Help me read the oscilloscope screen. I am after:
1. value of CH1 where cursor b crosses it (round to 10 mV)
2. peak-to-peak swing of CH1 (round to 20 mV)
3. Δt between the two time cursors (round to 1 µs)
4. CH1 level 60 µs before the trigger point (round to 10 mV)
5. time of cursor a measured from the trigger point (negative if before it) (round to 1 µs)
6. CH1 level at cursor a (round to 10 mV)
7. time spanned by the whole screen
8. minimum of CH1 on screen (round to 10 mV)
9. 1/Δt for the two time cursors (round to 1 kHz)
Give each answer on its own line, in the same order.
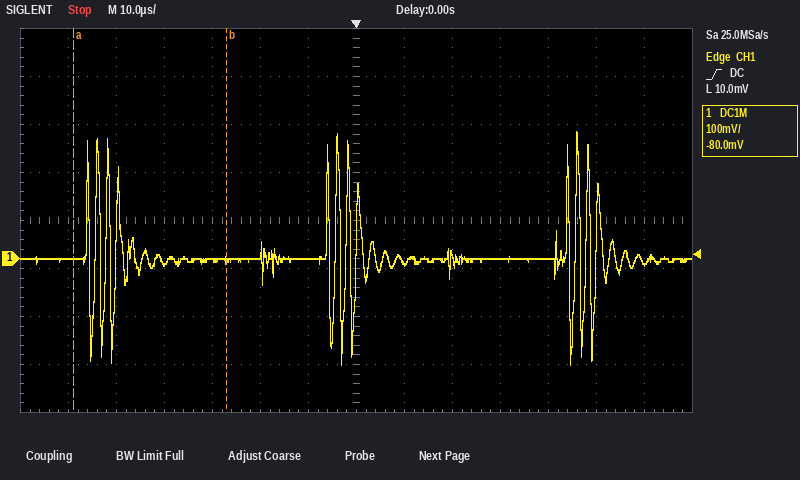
0 mV
480 mV
32 µs
0 mV
-59 µs
0 mV
140 µs
-220 mV
31 kHz
